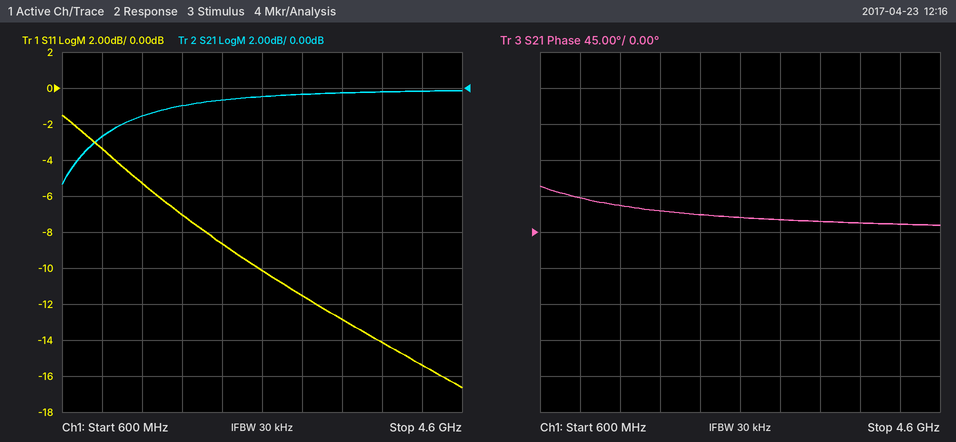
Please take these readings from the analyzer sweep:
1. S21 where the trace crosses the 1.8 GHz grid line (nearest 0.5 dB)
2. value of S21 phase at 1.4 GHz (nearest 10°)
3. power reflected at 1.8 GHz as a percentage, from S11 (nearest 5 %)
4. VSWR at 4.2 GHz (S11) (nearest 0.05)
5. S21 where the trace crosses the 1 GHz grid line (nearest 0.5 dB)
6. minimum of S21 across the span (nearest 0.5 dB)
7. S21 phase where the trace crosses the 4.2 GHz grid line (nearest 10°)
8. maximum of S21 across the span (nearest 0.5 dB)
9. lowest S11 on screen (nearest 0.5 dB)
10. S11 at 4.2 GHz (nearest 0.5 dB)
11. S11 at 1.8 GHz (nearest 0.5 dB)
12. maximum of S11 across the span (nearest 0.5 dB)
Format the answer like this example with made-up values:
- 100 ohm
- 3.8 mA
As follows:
- -1.0 dB
- 30°
- 20 %
- 1.40
- -2.5 dB
- -5.5 dB
- 10°
- 0.0 dB
- -16.5 dB
- -15.5 dB
- -7.0 dB
- -1.5 dB
